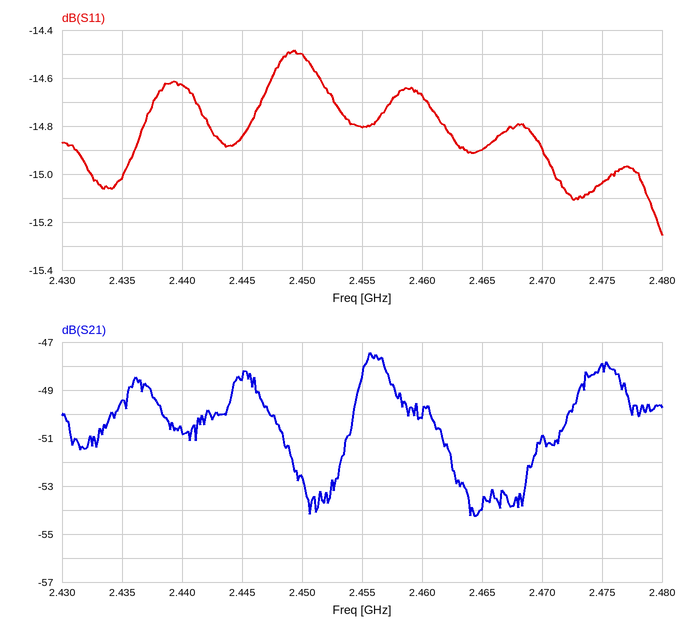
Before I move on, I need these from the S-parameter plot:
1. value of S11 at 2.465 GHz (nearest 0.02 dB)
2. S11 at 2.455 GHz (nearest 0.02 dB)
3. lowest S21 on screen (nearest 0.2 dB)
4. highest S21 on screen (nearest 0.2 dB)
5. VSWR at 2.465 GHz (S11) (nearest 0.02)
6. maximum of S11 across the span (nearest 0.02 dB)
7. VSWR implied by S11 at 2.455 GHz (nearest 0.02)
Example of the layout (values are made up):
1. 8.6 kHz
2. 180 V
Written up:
1. -14.90 dB
2. -14.80 dB
3. -54.2 dB
4. -47.4 dB
5. 1.44
6. -14.48 dB
7. 1.44
